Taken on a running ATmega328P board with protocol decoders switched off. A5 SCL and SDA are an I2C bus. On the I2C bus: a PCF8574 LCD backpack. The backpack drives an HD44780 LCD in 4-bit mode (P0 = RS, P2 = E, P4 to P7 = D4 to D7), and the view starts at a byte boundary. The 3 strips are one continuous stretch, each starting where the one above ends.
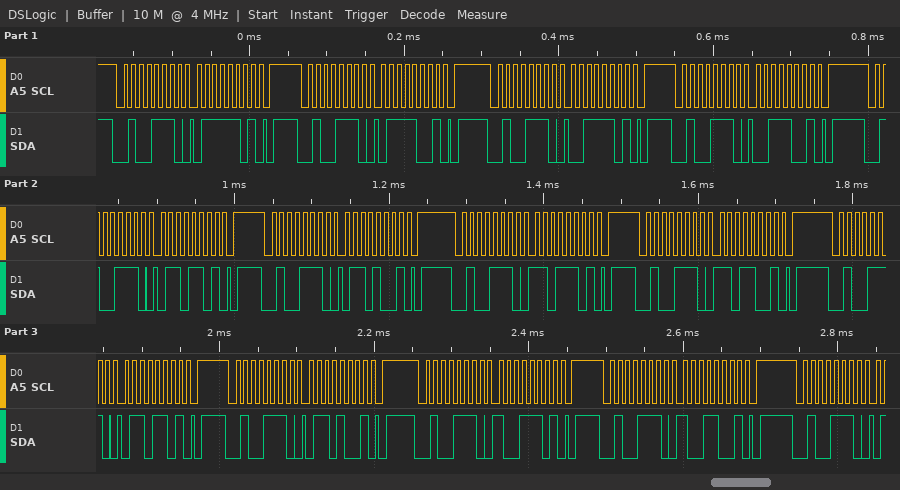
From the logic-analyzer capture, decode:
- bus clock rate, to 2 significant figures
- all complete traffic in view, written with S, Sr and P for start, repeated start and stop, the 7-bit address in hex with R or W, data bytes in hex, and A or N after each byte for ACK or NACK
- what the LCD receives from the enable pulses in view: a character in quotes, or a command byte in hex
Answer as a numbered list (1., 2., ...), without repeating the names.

1. 100 kHz
2. S 27W A 7D A P S 27W A 79 A P S 27W A 3D A P S 27W A 39 A P S 27W A 6D A P S 27W A 69 A P S 27W A DD A P S 27W A D9 A P S 27W A 6D A P S 27W A 69 A P S 27W A 9D A P S 27W A 99 A P S 27W A
3. 's' 'm' 'i'
